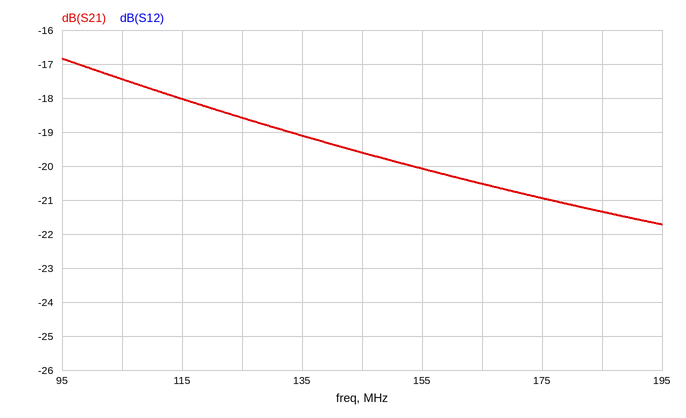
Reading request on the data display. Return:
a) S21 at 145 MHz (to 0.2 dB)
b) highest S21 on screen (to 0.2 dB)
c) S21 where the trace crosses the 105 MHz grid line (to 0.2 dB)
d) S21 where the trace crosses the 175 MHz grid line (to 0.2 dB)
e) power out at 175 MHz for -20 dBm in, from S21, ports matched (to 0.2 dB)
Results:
-19.6 dB
-16.8 dB
-17.4 dB
-21.0 dB
-41.0 dBm
